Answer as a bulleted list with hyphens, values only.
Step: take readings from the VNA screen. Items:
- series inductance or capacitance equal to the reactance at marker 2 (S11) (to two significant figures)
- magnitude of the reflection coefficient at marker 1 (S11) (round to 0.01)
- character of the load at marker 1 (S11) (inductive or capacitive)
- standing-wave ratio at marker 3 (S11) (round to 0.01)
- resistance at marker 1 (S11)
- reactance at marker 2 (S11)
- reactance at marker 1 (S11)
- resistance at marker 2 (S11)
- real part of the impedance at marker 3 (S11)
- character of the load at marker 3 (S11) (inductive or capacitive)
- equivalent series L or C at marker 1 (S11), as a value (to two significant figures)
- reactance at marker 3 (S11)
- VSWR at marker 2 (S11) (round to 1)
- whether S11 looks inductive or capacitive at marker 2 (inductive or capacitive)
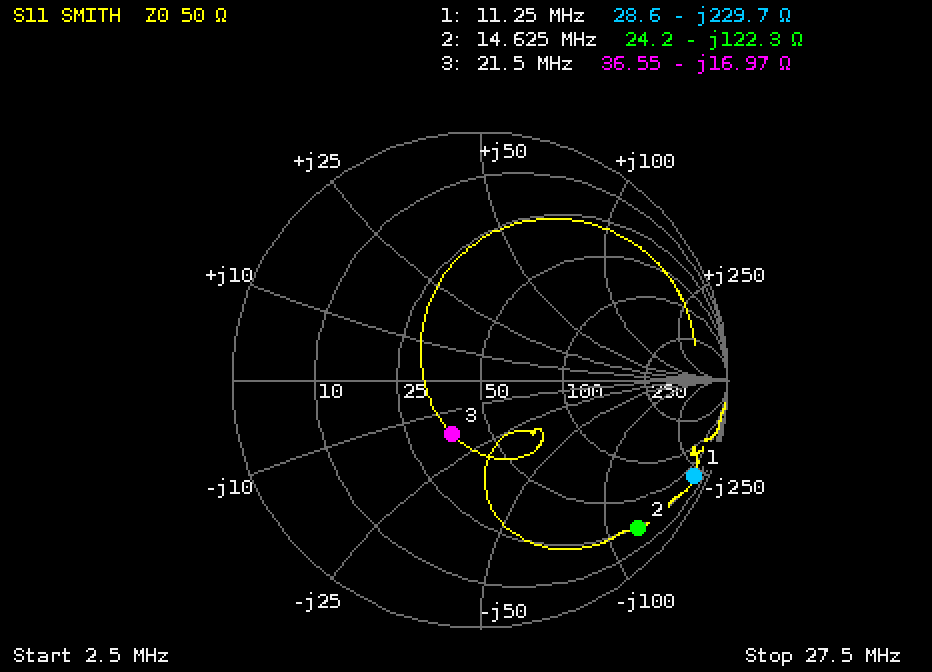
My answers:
- 89 pF
- 0.95
- capacitive
- 1.65
- 28.6 Ω
- -122.3 Ω
- -229.7 Ω
- 24.2 Ω
- 36.55 Ω
- capacitive
- 62 pF
- -16.97 Ω
- 15
- capacitive
